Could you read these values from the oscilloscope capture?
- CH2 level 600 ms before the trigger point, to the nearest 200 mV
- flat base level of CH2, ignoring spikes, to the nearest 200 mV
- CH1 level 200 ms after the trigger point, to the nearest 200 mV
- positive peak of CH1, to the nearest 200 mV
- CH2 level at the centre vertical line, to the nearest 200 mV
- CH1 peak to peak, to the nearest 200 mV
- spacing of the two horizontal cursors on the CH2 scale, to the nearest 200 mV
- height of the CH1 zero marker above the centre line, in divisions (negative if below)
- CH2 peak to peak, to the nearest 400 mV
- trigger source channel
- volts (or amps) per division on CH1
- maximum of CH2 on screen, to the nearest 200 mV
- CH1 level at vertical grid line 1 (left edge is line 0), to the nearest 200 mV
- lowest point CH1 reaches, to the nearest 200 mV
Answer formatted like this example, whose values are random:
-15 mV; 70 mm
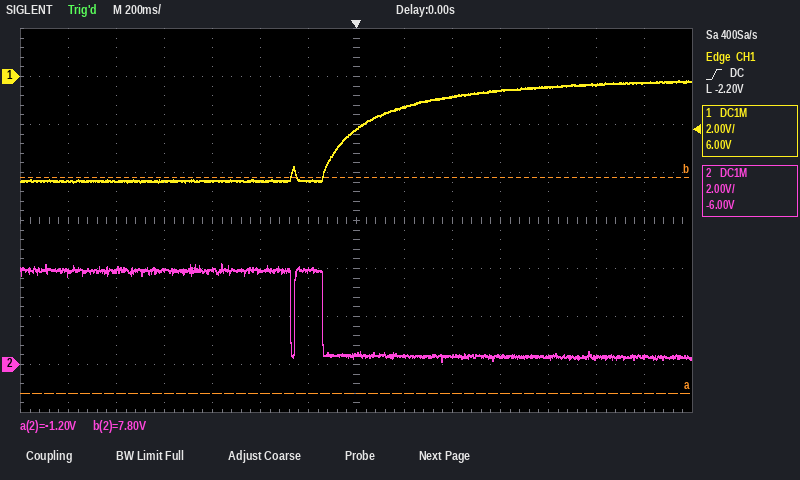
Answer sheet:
4.0 V; 400 mV; -1.2 V; -200 mV; 400 mV; 4.2 V; 9.0 V; +3.0 div; 4.0 V; CH1; 2 V; 4.2 V; -4.4 V; -4.4 V
